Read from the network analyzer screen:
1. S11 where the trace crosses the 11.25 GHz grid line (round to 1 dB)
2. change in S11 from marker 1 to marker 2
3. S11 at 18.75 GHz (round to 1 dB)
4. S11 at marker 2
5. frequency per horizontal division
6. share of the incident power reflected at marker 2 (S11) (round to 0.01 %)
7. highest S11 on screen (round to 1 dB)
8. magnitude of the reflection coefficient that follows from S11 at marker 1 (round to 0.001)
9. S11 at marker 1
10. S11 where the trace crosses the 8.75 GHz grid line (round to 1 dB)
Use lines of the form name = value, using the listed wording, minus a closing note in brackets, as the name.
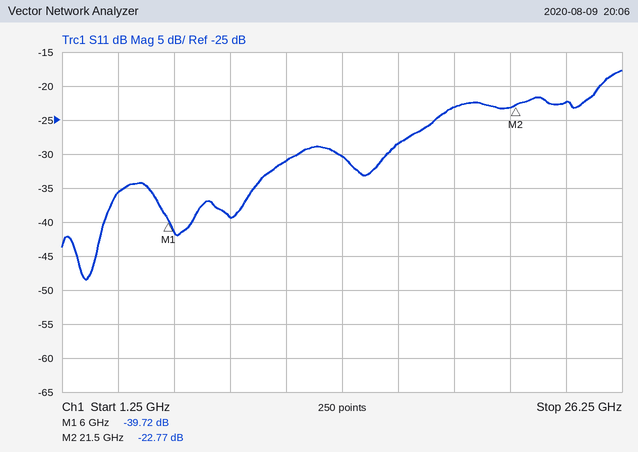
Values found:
S11 where the trace crosses the 11.25 GHz grid line = -31 dB
change in S11 from marker 1 to marker 2 = 16.95 dB
S11 at 18.75 GHz = -23 dB
S11 at marker 2 = -22.77 dB
frequency per horizontal division = 2.5 GHz
share of the incident power reflected at marker 2 (S11) = 0.53 %
highest S11 on screen = -18 dB
magnitude of the reflection coefficient that follows from S11 at marker 1 = 0.010
S11 at marker 1 = -39.72 dB
S11 where the trace crosses the 8.75 GHz grid line = -39 dB
